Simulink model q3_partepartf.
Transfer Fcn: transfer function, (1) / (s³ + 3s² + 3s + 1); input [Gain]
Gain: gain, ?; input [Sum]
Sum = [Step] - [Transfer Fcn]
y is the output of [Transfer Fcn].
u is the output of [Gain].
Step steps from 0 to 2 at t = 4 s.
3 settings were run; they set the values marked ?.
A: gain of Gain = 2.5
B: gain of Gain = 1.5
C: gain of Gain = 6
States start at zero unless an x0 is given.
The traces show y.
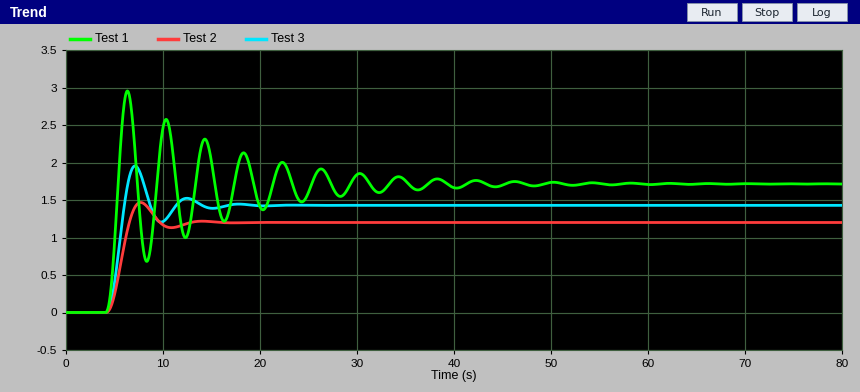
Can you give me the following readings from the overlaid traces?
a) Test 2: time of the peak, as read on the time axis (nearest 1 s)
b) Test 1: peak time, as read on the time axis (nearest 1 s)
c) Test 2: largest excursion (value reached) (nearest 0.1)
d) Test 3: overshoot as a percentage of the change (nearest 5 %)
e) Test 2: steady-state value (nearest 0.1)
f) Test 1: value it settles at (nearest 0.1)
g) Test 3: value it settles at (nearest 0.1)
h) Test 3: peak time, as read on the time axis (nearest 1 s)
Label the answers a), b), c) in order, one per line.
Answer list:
a) 8 s
b) 6 s
c) 1.5
d) 35 %
e) 1.2
f) 1.7
g) 1.4
h) 7 s
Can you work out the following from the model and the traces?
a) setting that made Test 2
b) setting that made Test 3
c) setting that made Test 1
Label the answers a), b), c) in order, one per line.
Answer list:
a) B
b) A
c) C
